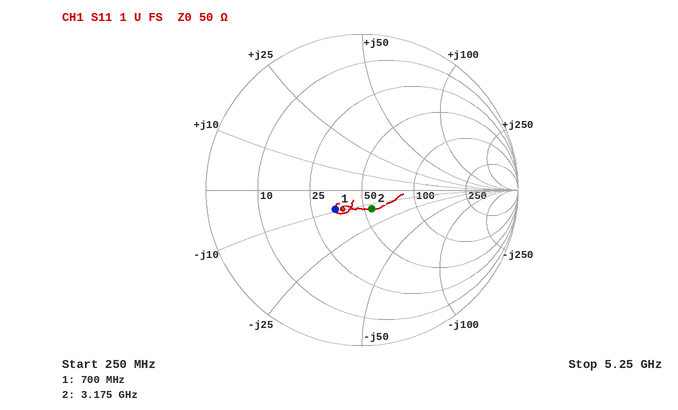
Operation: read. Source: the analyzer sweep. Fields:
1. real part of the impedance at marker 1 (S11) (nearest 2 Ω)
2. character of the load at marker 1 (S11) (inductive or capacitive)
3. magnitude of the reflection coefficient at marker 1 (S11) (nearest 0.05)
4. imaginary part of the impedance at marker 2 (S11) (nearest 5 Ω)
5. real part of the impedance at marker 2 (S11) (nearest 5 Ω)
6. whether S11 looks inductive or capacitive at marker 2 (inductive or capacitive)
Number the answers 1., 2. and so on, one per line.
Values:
1. 34 Ω
2. capacitive
3. 0.20
4. -15 Ω
5. 55 Ω
6. capacitive
